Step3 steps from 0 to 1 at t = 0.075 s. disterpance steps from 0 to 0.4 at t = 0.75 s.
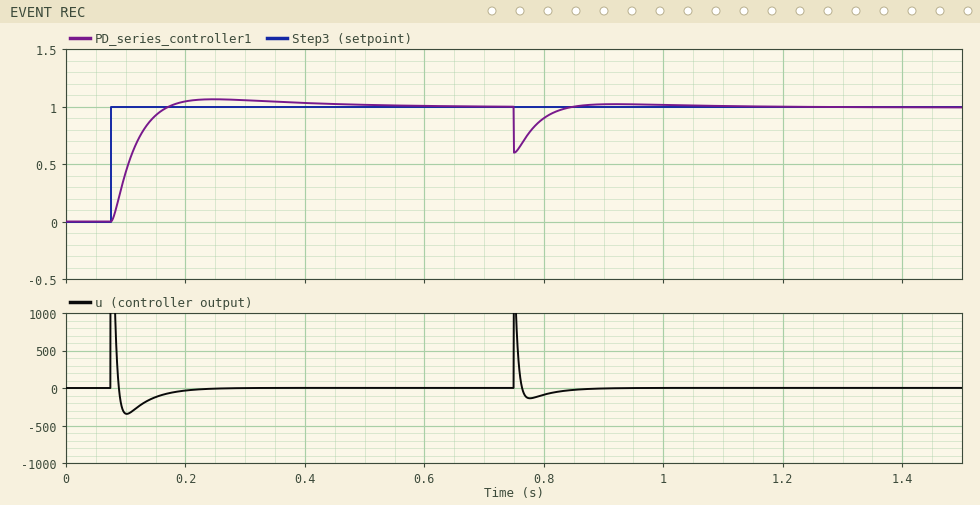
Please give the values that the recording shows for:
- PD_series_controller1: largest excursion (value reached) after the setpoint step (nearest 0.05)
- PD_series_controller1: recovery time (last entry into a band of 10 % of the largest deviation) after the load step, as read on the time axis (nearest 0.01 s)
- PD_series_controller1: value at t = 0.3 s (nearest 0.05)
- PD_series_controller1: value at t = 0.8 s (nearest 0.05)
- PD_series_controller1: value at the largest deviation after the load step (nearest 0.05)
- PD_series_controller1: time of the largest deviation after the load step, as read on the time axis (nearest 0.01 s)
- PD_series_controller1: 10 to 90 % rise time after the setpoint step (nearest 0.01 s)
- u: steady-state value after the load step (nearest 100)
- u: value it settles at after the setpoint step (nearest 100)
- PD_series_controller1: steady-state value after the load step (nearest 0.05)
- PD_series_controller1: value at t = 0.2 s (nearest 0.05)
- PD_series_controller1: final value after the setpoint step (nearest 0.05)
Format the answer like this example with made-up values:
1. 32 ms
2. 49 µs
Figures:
1. 1.05
2. 0.82 s
3. 1.05
4. 0.90
5. 0.60
6. 0.75 s
7. 0.06 s
8. 0
9. 0
10. 1.00
11. 1.05
12. 1.00
